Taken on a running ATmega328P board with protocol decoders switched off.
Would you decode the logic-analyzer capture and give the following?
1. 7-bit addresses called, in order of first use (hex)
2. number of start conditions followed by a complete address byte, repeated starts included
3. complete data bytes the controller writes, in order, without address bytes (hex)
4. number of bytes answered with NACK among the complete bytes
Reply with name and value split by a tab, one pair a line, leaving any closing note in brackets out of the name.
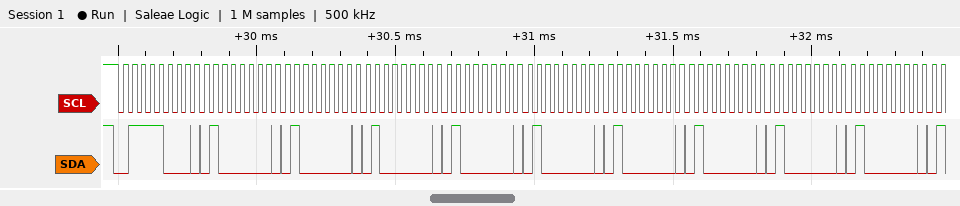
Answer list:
7-bit addresses called, in order of first use	0x3C
number of start conditions followed by a complete address byte, repeated starts included	1
complete data bytes the controller writes, in order, without address bytes	40 40 40 40 40 40 40 40 40
number of bytes answered with NACK among the complete bytes	0
